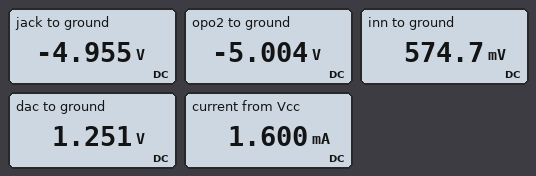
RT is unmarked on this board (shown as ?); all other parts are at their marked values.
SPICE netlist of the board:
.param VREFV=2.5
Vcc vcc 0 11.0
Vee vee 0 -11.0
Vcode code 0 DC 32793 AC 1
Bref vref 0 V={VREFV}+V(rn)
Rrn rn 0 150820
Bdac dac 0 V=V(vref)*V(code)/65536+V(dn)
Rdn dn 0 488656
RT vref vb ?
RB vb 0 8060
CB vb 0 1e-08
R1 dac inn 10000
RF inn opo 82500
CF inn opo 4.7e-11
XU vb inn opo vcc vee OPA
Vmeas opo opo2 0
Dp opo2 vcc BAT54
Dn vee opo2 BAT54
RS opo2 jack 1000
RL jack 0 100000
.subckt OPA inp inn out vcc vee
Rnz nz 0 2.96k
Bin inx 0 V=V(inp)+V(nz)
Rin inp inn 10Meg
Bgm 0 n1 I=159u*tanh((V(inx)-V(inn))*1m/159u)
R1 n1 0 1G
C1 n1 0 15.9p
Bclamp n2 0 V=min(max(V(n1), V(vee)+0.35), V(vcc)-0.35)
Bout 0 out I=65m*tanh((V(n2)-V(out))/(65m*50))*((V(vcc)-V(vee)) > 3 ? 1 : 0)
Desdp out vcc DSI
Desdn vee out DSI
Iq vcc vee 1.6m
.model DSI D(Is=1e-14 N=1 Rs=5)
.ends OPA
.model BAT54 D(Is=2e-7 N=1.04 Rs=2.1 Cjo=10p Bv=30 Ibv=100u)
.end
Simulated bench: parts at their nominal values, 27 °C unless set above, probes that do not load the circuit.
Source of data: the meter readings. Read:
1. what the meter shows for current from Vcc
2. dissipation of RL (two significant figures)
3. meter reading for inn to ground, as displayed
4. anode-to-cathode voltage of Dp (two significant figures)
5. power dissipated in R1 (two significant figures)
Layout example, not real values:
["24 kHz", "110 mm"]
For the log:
["1.600 mA", "250 µW", "574.7 mV", "-16 V", "46 µW"]
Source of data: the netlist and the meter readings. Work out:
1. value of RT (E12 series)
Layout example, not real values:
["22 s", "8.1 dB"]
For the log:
["27 kΩ"]
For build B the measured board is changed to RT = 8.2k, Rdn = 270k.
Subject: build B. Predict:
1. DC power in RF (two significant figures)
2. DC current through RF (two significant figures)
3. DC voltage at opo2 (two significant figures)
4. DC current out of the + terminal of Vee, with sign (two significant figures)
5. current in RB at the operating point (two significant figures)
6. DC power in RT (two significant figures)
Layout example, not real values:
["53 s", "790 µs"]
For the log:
["110 nW", "1.2 µA", "1.1 V", "-1.6 mA", "150 µA", "190 µW"]
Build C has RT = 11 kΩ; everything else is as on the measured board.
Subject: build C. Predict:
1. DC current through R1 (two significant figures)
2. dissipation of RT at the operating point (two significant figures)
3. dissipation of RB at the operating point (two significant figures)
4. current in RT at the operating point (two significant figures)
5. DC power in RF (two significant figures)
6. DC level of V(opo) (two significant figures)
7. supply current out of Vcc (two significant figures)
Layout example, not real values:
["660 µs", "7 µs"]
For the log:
["19 µA", "190 µW", "140 µW", "130 µA", "31 µW", "-540 mV", "1.6 mA"]
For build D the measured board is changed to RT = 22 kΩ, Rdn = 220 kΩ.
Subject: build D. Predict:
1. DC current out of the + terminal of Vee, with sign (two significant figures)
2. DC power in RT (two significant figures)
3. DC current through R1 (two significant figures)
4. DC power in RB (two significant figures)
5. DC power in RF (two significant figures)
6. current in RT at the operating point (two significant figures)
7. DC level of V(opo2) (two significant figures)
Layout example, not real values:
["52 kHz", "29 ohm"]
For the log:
["-1.6 mA", "150 µW", "58 µA", "56 µW", "280 µW", "83 µA", "-4.1 V"]
